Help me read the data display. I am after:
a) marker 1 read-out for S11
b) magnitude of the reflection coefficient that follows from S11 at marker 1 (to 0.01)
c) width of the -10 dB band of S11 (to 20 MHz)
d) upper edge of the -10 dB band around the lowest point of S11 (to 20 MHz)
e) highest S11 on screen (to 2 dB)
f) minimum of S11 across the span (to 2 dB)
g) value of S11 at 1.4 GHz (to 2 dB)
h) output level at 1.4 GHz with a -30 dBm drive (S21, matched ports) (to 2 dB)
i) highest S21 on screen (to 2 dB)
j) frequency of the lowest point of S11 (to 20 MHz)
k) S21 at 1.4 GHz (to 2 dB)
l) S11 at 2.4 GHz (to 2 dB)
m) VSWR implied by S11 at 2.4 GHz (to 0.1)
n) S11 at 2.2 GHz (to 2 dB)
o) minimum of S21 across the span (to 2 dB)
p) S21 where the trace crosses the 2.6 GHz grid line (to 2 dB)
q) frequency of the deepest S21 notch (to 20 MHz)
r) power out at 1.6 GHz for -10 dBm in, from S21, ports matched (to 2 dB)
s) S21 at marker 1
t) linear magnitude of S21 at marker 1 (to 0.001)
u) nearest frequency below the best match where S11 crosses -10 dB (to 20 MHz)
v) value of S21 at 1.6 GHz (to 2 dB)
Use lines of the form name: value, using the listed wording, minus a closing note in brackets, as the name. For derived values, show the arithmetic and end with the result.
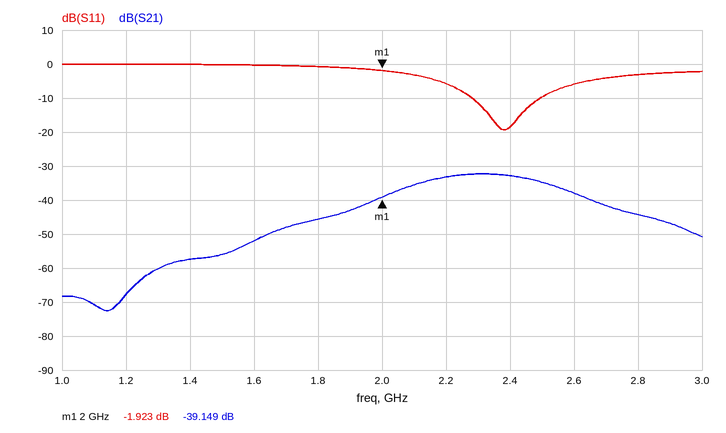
marker 1 read-out for S11: -1.923 dB
magnitude of the reflection coefficient that follows from S11 at marker 1: 10^(-1.923/20) ≈ 0.80
width of the -10 dB band of S11: 2.50 GHz − 2.28 GHz = 220 MHz
upper edge of the -10 dB band around the lowest point of S11: 2.50 GHz
highest S11 on screen: 0 dB
minimum of S11 across the span: -20 dB
value of S11 at 1.4 GHz: 0 dB
output level at 1.4 GHz with a -30 dBm drive (S21, matched ports): -30 dBm + (-58 dB) = -88 dBm
highest S21 on screen: -32 dB
frequency of the lowest point of S11: 2.38 GHz
S21 at 1.4 GHz: -58 dB
S11 at 2.4 GHz: -18 dB
VSWR implied by S11 at 2.4 GHz: |Γ| = 10^(-18/20) = 0.1259; VSWR = (1 + 0.1259)/(1 − 0.1259) ≈ 1.3
S11 at 2.2 GHz: -6 dB
minimum of S21 across the span: -72 dB
S21 where the trace crosses the 2.6 GHz grid line: -38 dB
frequency of the deepest S21 notch: 1.14 GHz
power out at 1.6 GHz for -10 dBm in, from S21, ports matched: -10 dBm + (-52 dB) = -62 dBm
S21 at marker 1: -39.149 dB
linear magnitude of S21 at marker 1: 10^(-39.149/20) ≈ 0.011
nearest frequency below the best match where S11 crosses -10 dB: 2.28 GHz
value of S21 at 1.6 GHz: -52 dB
